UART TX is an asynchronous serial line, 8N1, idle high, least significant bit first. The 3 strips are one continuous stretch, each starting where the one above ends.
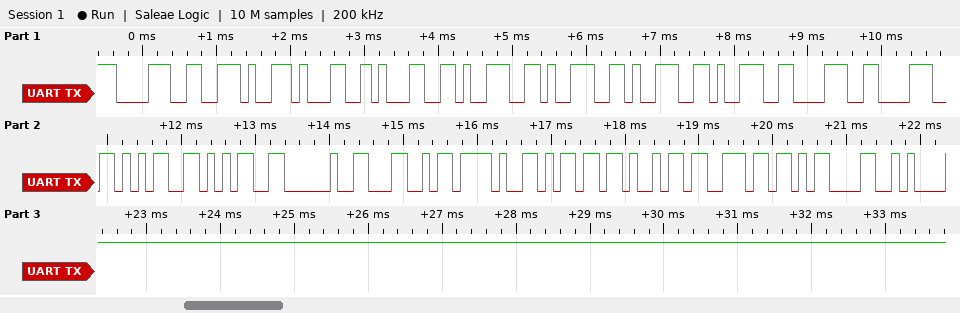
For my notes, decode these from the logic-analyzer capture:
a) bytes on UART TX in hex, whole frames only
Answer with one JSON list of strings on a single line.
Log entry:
["0x38 0x2E 0x31 0x31 0x39 0x39 0x39 0x39 0x38 0x38 0x35 0x35 0x20 0x4C 0x2F 0x6D 0x69 0x6E 0x0D 0x0A"]
